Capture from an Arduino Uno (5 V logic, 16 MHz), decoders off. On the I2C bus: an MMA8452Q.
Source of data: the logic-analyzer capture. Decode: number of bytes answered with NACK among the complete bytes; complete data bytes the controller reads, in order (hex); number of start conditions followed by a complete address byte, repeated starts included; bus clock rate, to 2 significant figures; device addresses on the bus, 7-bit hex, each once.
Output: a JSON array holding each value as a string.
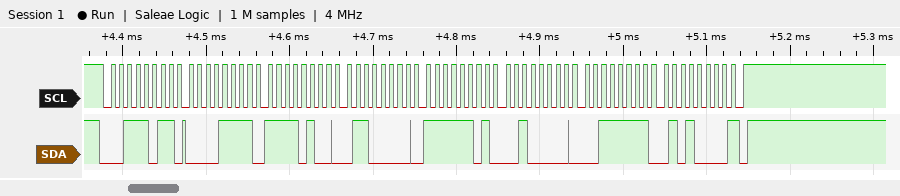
["1", "0F F4 60 FD 20 3F 50", "1", "100 kHz", "0x1D"]
